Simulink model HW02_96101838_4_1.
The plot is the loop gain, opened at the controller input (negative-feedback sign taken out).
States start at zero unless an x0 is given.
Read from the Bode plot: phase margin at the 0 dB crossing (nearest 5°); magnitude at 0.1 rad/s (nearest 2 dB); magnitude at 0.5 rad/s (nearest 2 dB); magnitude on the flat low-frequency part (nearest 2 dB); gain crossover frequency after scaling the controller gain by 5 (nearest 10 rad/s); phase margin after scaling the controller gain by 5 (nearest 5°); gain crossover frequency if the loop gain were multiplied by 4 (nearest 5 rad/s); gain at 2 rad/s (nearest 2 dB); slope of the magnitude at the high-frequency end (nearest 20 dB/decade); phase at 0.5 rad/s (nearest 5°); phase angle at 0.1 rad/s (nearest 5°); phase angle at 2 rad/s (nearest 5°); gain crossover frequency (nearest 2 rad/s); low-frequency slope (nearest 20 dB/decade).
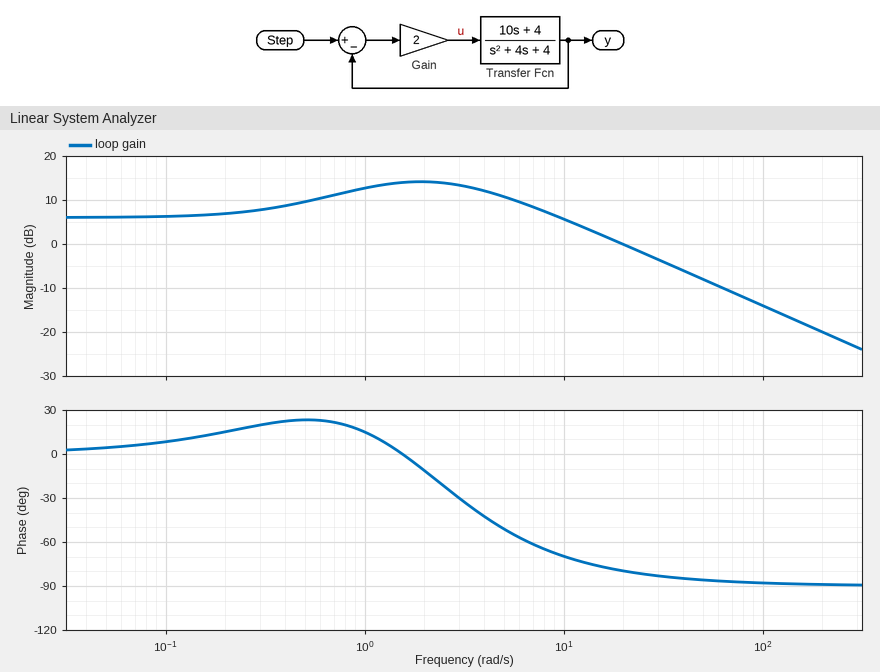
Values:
100°
6 dB
10 dB
6 dB
100 rad/s
90°
80 rad/s
14 dB
-20 dB/decade
25°
10°
-10°
20 rad/s
0 dB/decade
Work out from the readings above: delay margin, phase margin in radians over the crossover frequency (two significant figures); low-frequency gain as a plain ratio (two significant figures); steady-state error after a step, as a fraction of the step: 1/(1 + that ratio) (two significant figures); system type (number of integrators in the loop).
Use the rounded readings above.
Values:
0.087 s
2.0
0.33
0
